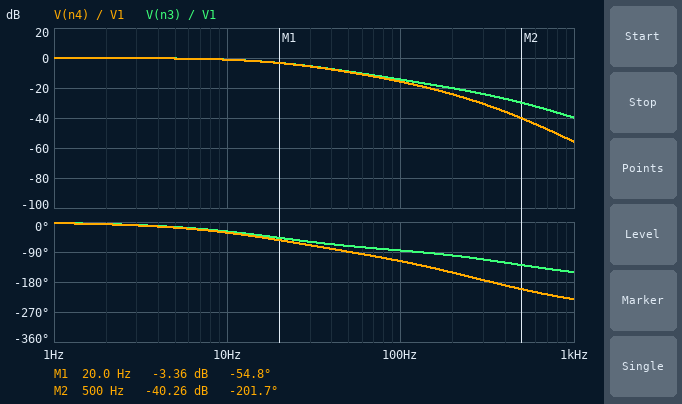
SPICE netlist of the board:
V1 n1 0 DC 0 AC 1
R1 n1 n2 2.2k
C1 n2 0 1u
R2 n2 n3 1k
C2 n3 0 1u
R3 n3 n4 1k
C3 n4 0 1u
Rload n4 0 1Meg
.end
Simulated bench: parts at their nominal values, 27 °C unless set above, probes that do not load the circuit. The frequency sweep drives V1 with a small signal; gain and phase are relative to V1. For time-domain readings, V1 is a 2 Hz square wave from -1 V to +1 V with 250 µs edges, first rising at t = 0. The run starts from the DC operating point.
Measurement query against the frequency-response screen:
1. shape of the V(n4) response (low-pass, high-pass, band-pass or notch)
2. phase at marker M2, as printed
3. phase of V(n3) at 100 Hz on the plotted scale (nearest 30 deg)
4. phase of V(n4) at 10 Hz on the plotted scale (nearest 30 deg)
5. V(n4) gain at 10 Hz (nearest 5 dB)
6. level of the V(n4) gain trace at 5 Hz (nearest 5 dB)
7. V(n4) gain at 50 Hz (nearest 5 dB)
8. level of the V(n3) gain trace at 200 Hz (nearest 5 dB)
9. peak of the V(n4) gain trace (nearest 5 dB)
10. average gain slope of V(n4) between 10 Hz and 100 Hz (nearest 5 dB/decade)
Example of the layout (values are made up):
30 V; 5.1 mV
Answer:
low-pass; -201.7 deg; -90 deg; -30 deg; 0 dB; 0 dB; -10 dB; -20 dB; 0 dB; -15 dB/decade
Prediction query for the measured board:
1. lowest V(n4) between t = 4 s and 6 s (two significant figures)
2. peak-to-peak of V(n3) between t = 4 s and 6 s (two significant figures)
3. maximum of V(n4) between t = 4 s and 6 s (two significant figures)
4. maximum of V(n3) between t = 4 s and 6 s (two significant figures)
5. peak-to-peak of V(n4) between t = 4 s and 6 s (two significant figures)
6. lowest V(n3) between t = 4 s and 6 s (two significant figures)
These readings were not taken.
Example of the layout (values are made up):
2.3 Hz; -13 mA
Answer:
-1.0 V; 2.0 V; 1.0 V; 1.0 V; 2.0 V; -1.0 V
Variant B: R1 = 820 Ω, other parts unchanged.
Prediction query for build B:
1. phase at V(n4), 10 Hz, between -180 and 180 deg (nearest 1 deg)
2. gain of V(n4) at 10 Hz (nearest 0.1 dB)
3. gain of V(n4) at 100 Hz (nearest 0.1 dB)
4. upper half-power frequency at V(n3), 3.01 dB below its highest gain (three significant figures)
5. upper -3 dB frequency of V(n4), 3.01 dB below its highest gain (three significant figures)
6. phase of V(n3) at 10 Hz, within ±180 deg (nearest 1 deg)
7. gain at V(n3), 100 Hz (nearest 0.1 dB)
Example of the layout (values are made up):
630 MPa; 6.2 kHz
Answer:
-19 deg; -0.4 dB; -10.4 dB; 35.9 Hz; 34.3 Hz; -16 deg; -8.9 dB
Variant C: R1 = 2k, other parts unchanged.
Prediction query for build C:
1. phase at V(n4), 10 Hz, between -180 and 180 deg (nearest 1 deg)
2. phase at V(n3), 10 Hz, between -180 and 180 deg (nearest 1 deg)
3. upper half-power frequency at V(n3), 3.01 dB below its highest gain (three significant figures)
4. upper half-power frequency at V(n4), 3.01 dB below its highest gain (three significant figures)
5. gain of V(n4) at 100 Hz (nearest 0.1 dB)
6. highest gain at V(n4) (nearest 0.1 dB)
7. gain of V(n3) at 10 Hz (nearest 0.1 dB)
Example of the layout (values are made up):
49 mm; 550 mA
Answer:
-30 deg; -27 deg; 20.3 Hz; 20.0 Hz; -15.2 dB; 0 dB; -1.0 dB
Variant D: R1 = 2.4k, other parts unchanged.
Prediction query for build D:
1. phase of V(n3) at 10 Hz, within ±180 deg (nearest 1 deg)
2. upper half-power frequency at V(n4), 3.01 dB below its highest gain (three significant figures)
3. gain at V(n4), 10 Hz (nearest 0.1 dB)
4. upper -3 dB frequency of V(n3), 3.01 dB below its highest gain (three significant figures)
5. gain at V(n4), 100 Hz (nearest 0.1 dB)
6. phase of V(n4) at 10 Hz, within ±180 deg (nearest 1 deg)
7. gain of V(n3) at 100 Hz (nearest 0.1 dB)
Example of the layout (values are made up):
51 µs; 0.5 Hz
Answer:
-30 deg; 17.5 Hz; -1.3 dB; 17.7 Hz; -16.4 dB; -34 deg; -15.0 dB
